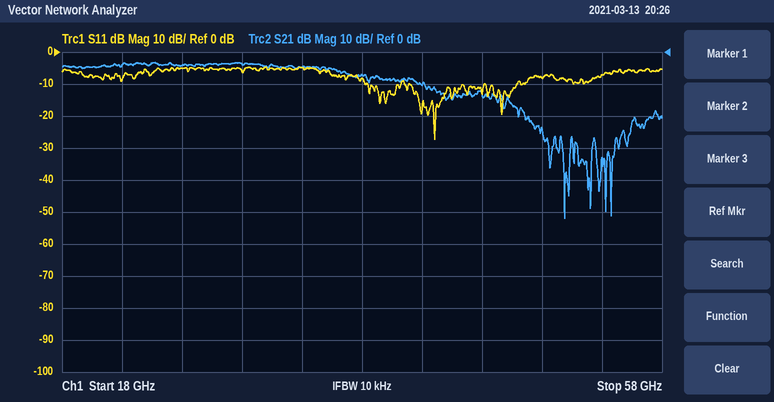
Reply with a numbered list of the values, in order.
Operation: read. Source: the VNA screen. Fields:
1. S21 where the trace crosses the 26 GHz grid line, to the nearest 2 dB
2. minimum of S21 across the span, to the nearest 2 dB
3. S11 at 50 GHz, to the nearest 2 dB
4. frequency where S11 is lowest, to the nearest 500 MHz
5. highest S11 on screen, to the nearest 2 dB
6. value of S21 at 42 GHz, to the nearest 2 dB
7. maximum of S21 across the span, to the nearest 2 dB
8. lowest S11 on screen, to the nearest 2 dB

1. -4 dB
2. -52 dB
3. -8 dB
4. 43.0 GHz
5. -4 dB
6. -10 dB
7. -4 dB
8. -28 dB
